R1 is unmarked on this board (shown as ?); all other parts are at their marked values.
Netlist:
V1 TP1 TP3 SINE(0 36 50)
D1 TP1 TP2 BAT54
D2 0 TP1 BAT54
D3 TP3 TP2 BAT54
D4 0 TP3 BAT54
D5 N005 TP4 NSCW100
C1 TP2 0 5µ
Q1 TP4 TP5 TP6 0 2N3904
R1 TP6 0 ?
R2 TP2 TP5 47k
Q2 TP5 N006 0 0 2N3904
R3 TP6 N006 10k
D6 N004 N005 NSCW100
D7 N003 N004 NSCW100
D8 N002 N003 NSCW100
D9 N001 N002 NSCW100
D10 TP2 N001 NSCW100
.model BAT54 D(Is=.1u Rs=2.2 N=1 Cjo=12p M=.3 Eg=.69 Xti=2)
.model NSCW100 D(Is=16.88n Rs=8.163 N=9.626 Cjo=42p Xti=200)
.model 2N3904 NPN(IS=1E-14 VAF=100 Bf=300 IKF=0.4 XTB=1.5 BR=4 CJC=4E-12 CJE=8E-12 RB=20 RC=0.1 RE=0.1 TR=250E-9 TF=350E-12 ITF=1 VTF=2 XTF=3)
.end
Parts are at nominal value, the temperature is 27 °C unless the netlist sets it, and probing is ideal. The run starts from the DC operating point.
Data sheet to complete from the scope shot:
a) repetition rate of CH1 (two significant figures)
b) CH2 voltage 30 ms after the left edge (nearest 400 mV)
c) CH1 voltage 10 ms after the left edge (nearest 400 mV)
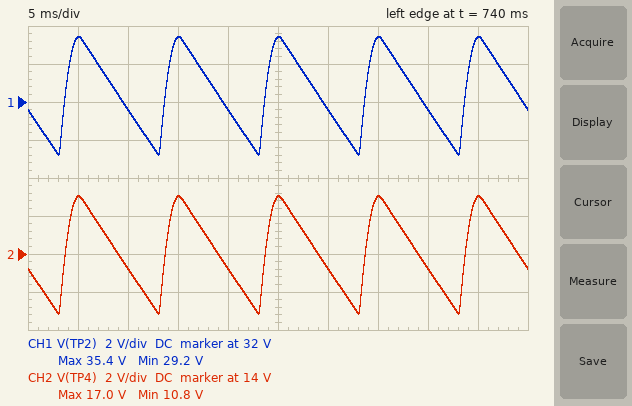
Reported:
100 Hz
13.2 V
31.6 V
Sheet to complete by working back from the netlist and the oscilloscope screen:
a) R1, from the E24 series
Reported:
200 Ω
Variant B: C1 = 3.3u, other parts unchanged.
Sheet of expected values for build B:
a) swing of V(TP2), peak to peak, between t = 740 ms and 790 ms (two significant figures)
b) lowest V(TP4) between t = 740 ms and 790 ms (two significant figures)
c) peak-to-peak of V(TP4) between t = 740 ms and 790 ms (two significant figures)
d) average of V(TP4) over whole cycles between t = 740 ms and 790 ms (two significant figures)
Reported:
8.9 V
8.2 V
8.8 V
13 V
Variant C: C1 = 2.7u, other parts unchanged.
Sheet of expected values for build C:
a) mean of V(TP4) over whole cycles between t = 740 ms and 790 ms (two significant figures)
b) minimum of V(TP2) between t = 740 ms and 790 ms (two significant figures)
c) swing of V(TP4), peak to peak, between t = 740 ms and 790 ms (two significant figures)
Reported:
12 V
25 V
10 V
